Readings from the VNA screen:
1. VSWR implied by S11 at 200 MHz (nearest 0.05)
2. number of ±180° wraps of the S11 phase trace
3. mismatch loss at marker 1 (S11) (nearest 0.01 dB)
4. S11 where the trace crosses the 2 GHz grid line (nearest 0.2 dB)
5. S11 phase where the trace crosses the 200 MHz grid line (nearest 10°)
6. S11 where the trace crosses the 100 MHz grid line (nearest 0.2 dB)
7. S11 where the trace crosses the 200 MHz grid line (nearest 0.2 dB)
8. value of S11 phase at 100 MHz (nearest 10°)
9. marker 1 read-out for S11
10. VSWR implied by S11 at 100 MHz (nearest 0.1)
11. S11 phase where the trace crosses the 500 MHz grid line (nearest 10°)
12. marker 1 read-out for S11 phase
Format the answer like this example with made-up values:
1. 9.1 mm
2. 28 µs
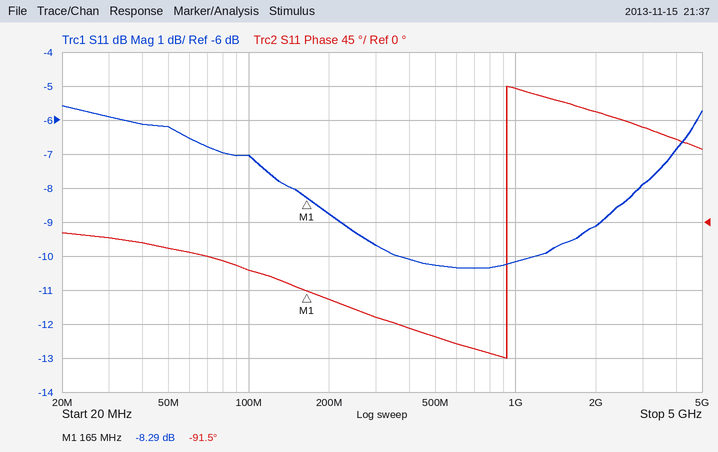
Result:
1. 2.15
2. 1
3. 0.70 dB
4. -9.2 dB
5. -100°
6. -7.0 dB
7. -8.8 dB
8. -60°
9. -8.29 dB
10. 2.6
11. -150°
12. -91.5°
